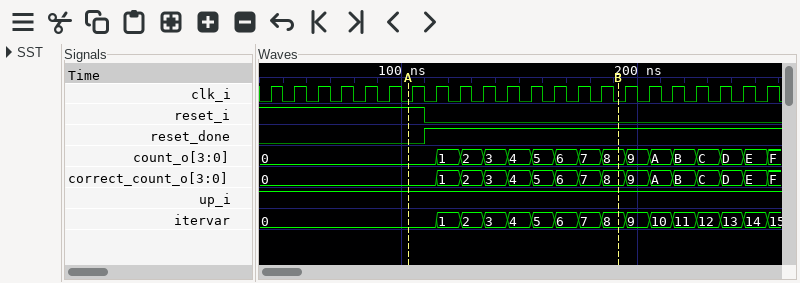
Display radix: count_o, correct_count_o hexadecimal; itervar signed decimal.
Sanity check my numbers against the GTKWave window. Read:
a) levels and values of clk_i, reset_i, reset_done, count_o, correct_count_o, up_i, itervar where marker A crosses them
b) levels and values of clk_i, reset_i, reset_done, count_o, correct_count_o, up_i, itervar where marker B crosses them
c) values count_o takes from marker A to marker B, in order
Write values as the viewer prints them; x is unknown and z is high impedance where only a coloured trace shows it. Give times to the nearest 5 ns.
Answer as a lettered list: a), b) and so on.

a) clk_i=0, reset_i=1, reset_done=0, count_o=0, correct_count_o=0, up_i=1, itervar=0
b) clk_i=0, reset_i=0, reset_done=1, count_o=8, correct_count_o=8, up_i=1, itervar=8
c) 0, 1, 2, 3, 4, 5, 6, 7, 8
